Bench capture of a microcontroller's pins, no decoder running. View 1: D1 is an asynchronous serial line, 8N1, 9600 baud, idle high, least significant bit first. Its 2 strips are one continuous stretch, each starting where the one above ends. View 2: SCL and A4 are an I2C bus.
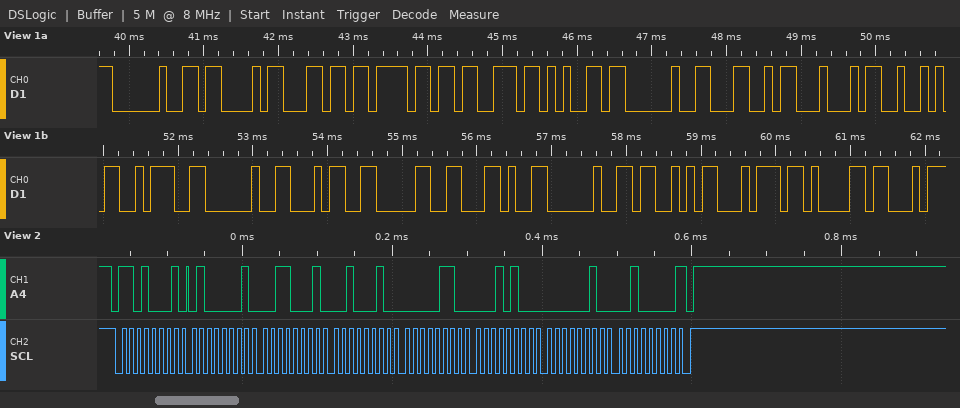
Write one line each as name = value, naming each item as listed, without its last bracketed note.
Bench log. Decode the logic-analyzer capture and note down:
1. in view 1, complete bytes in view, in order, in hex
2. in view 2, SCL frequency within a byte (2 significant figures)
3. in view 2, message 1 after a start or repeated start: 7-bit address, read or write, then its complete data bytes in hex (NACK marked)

in view 1, complete bytes in view, in order, in hex = 20 43 6C 6F 73 65 20 4C 44 52 3A 20 34 30 2C 20 53 74 61
in view 2, SCL frequency within a byte = 100 kHz
in view 2, message 1 after a start or repeated start: 7-bit address, read or write, then its complete data bytes in hex = 0x68 read: 41 31 22 06 14 02 20 NACK
